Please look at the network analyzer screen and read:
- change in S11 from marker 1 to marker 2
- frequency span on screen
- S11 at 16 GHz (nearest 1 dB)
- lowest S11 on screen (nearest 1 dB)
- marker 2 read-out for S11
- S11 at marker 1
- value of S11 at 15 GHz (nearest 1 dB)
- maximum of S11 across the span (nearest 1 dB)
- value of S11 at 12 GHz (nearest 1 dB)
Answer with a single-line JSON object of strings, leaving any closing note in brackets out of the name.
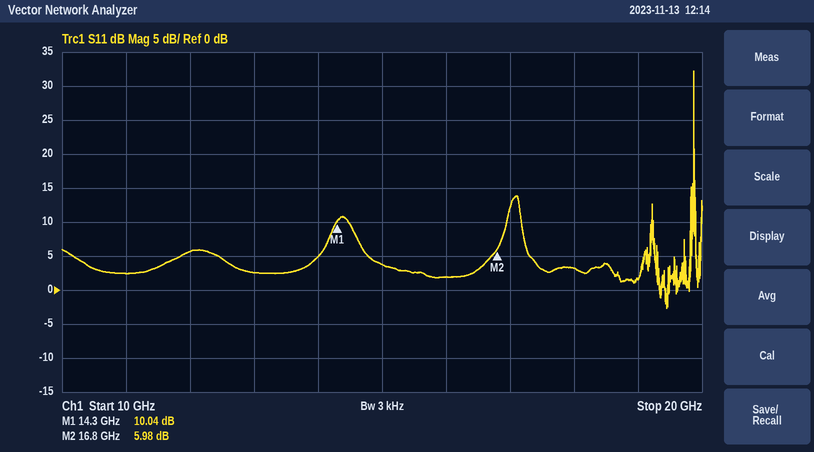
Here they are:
{"change in S11 from marker 1 to marker 2": "-4.06 dB", "frequency span on screen": "10 GHz", "S11 at 16 GHz": "2 dB", "lowest S11 on screen": "-3 dB", "marker 2 read-out for S11": "5.98 dB", "S11 at marker 1": "10.04 dB", "value of S11 at 15 GHz": "4 dB", "maximum of S11 across the span": "32 dB", "value of S11 at 12 GHz": "6 dB"}
